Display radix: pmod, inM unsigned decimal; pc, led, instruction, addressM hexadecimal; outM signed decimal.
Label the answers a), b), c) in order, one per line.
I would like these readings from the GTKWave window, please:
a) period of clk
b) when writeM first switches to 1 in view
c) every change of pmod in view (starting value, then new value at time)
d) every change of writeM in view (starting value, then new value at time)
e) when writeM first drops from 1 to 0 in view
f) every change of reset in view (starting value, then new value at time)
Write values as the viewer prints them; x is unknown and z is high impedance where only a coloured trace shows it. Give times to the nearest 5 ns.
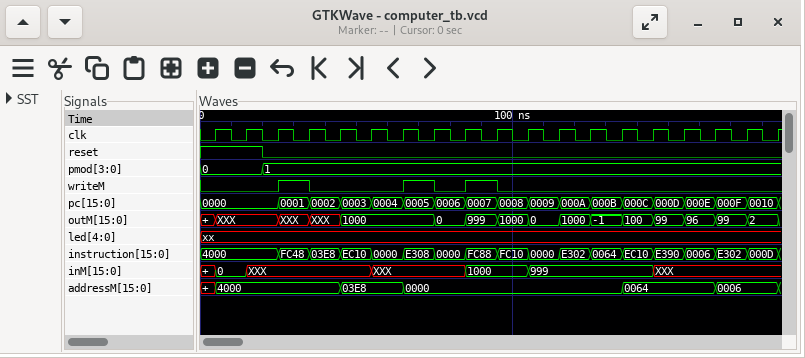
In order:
a) 10 ns
b) 25 ns
c) 0, 1 at 20 ns
d) 0, 1 at 25 ns, 0 at 35 ns, 1 at 65 ns, 0 at 75 ns, 1 at 85 ns, 0 at 95 ns
e) 35 ns
f) 1, 0 at 20 ns
